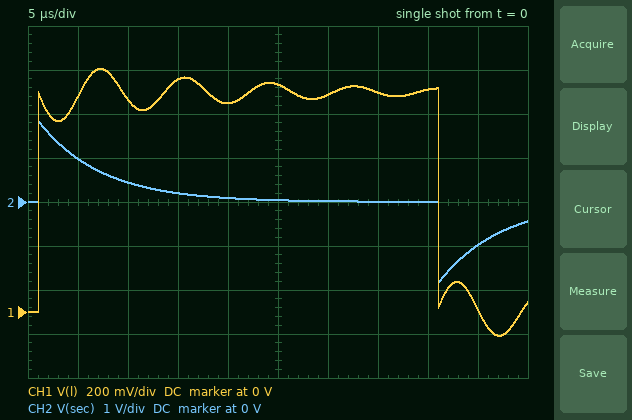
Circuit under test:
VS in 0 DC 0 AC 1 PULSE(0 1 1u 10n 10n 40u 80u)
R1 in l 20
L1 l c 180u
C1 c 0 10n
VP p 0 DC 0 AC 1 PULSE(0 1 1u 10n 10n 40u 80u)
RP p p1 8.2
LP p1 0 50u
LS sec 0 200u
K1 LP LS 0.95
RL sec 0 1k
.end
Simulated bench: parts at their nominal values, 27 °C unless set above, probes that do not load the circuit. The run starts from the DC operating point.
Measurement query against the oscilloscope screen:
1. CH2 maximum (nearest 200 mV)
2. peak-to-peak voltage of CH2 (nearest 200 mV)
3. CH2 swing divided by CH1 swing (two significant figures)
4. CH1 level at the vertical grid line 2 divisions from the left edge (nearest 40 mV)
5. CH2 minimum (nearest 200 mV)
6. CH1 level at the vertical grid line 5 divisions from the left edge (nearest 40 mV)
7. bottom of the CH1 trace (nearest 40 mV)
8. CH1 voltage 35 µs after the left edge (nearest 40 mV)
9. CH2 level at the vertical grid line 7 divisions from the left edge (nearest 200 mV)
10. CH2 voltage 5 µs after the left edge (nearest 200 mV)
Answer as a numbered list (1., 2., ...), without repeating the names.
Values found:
1. 1.8 V
2. 3.6 V
3. 3.0
4. 960 mV
5. -1.8 V
6. 1.04 V
7. -120 mV
8. 1.00 V
9. 0 V
10. 1.0 V
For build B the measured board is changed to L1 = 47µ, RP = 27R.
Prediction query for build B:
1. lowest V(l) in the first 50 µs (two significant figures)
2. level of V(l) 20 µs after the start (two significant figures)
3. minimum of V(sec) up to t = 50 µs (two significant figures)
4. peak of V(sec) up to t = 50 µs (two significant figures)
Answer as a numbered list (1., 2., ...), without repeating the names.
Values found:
1. -150 mV
2. 1.0 V
3. -1.7 V
4. 1.7 V
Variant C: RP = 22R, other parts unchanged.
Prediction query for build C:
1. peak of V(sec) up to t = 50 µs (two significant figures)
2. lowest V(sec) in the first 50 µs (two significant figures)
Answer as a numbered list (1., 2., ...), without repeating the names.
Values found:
1. 1.7 V
2. -1.7 V
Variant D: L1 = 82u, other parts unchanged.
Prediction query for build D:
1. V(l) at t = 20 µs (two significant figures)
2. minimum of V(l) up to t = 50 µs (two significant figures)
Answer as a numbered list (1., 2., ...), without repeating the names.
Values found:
1. 980 mV
2. -130 mV
